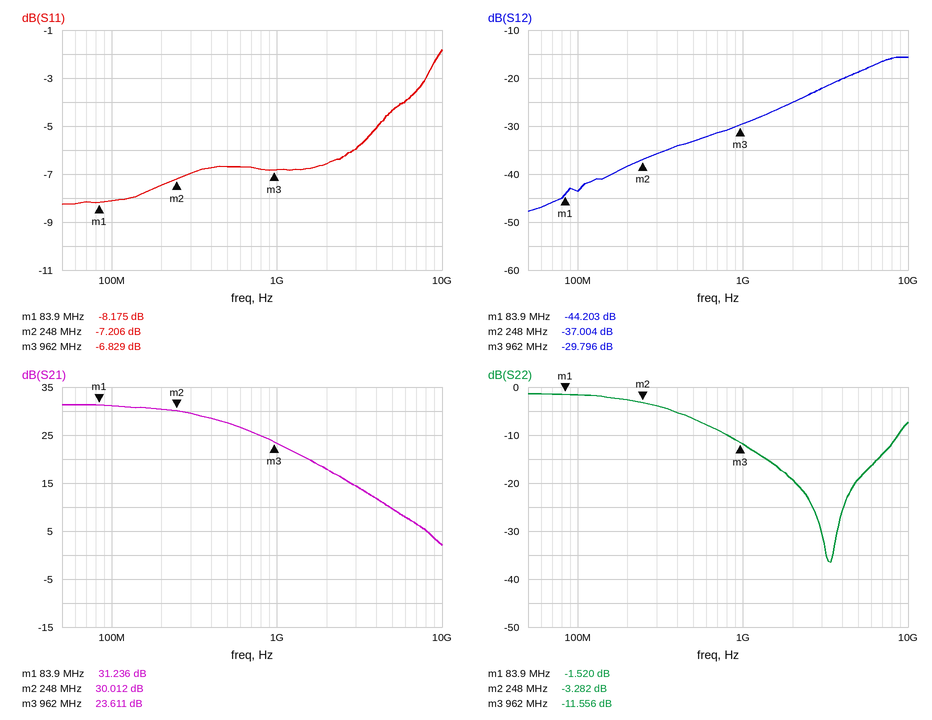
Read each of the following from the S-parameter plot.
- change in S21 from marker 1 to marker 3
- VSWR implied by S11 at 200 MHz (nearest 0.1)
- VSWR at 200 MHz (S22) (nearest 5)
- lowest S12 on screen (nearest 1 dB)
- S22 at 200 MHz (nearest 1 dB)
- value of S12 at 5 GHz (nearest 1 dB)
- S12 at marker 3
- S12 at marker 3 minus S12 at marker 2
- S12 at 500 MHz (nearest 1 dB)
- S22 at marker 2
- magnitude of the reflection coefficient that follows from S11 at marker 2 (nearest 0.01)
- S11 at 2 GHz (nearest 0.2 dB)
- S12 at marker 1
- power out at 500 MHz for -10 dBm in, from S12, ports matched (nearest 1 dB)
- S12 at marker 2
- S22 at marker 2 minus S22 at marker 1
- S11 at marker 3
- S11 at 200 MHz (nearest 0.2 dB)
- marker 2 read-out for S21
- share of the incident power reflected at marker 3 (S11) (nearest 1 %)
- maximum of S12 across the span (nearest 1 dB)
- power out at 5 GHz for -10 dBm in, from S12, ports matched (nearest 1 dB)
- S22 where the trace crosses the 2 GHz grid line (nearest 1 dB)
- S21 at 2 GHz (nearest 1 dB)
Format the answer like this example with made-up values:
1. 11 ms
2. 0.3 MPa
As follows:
1. -7.625 dB
2. 2.5
3. 5
4. -48 dB
5. -3 dB
6. -19 dB
7. -29.796 dB
8. 7.208 dB
9. -33 dB
10. -3.282 dB
11. 0.44
12. -6.6 dB
13. -44.203 dB
14. -43 dBm
15. -37.004 dB
16. -1.762 dB
17. -6.829 dB
18. -7.4 dB
19. 30.012 dB
20. 21 %
21. -16 dB
22. -29 dBm
23. -19 dB
24. 18 dB
